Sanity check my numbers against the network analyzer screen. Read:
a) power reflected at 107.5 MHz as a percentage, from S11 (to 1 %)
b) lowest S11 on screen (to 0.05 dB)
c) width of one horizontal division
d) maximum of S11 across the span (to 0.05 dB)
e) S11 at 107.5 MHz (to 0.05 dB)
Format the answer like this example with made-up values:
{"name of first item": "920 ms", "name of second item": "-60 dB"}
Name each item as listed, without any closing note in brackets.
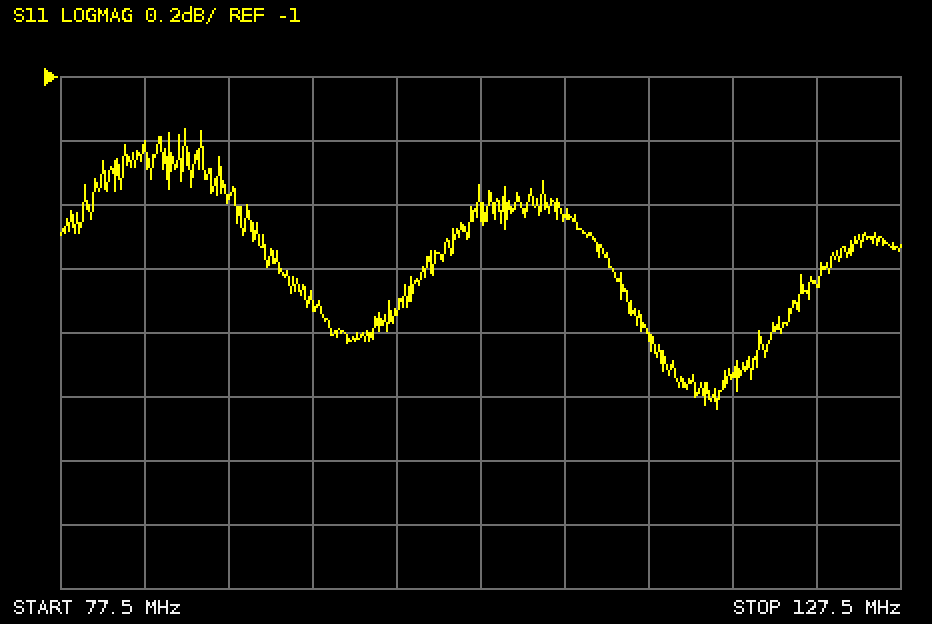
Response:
{"power reflected at 107.5 MHz as a percentage, from S11": "72 %", "lowest S11 on screen": "-2.05 dB", "width of one horizontal division": "5 MHz", "maximum of S11 across the span": "-1.15 dB", "S11 at 107.5 MHz": "-1.45 dB"}
